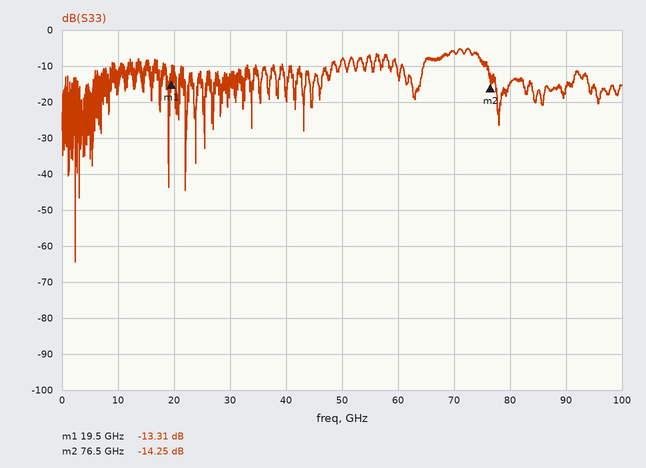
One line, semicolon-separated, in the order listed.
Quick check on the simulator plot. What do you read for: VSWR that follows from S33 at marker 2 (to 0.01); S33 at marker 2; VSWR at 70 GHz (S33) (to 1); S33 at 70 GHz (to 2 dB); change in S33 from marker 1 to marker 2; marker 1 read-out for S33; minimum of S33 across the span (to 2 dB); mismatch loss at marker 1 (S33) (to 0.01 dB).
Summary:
1.48; -14.25 dB; 3; -6 dB; -0.94 dB; -13.31 dB; -64 dB; 0.21 dB
